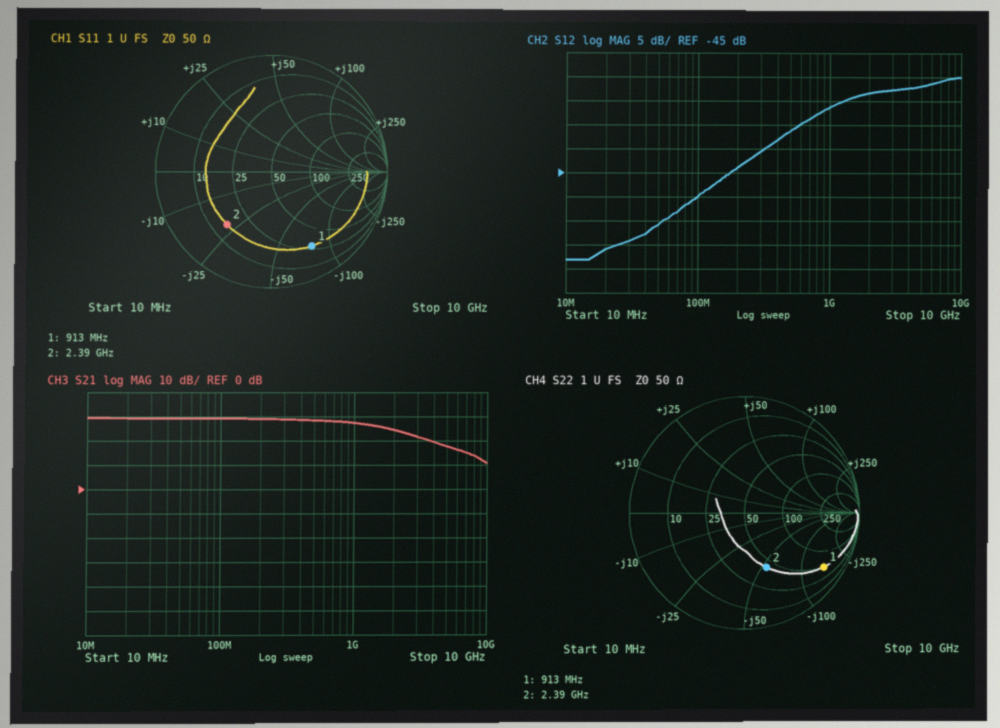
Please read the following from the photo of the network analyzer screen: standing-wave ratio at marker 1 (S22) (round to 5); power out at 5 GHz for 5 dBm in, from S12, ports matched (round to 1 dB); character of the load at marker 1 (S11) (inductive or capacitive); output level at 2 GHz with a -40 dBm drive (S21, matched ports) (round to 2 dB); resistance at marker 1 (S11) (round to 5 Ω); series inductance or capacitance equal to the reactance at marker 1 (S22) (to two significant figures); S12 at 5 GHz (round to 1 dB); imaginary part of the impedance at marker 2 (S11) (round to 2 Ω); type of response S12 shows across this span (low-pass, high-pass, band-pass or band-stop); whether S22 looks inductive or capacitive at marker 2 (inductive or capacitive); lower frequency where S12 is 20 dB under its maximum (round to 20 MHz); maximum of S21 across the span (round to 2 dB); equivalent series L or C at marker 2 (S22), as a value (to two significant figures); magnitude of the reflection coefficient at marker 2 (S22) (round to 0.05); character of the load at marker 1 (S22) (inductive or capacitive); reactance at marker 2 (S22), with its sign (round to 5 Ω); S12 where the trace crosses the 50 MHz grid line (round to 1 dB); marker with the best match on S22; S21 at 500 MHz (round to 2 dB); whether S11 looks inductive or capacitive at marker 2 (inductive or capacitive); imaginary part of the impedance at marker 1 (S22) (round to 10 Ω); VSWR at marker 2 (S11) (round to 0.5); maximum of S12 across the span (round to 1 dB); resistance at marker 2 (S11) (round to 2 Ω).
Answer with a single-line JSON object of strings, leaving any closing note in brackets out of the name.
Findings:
{"standing-wave ratio at marker 1 (S22)": "10", "power out at 5 GHz for 5 dBm in, from S12, ports matched": "-22 dBm", "character of the load at marker 1 (S11)": "capacitive", "output level at 2 GHz with a -40 dBm drive (S21, matched ports)": "-16 dBm", "resistance at marker 1 (S11)": "30 Ω", "series inductance or capacitance equal to the reactance at marker 1 (S22)": "1.2 pF", "S12 at 5 GHz": "-27 dB", "imaginary part of the impedance at marker 2 (S11)": "-22 Ω", "type of response S12 shows across this span": "high-pass", "whether S22 looks inductive or capacitive at marker 2": "capacitive", "lower frequency where S12 is 20 dB under its maximum": "180 MHz", "maximum of S21 across the span": "30 dB", "equivalent series L or C at marker 2 (S22), as a value": "1.2 pF", "magnitude of the reflection coefficient at marker 2 (S22)": "0.50", "character of the load at marker 1 (S22)": "capacitive", "reactance at marker 2 (S22), with its sign": "-55 Ω", "S12 where the trace crosses the 50 MHz grid line": "-56 dB", "marker with the best match on S22": "marker 2", "S21 at 500 MHz": "28 dB", "whether S11 looks inductive or capacitive at marker 2": "capacitive", "imaginary part of the impedance at marker 1 (S22)": "-150 Ω", "VSWR at marker 2 (S11)": "4.0", "maximum of S12 across the span": "-25 dB", "resistance at marker 2 (S11)": "16 Ω"}
